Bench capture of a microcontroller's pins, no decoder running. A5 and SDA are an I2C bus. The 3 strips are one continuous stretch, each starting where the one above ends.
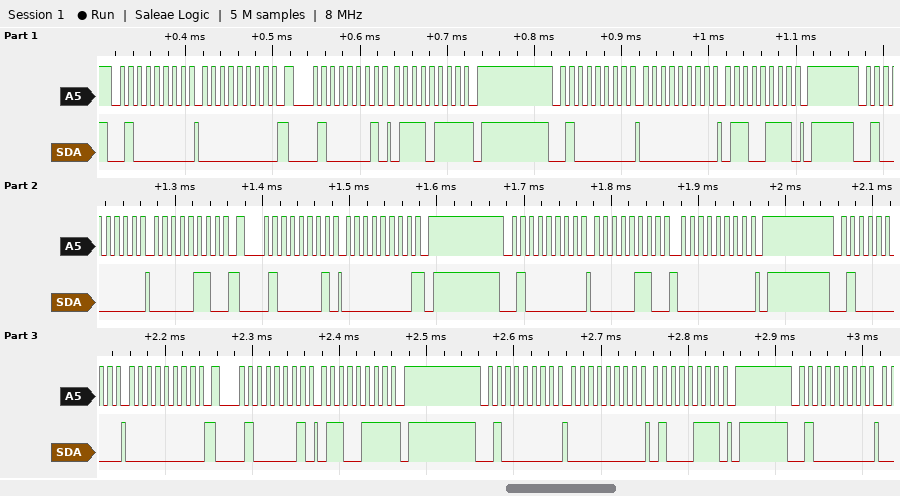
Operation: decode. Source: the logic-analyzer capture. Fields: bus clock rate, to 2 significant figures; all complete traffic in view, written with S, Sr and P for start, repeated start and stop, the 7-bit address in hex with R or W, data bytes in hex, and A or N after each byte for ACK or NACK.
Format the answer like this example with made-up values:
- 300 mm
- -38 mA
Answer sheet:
- 100 kHz
- S 20W A 00 A Sr 20R A 77 N P S 20W A 00 A 67 A P S 20W A 06 A Sr 20R A 00 N P S 20W A 06 A 00 A P S 20W A 00 A Sr 20R A 67 N P S 20W A 00 A 47 A P S 20W A
